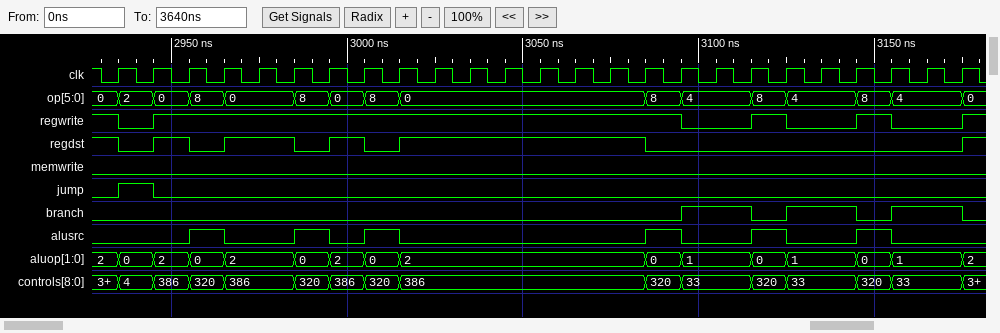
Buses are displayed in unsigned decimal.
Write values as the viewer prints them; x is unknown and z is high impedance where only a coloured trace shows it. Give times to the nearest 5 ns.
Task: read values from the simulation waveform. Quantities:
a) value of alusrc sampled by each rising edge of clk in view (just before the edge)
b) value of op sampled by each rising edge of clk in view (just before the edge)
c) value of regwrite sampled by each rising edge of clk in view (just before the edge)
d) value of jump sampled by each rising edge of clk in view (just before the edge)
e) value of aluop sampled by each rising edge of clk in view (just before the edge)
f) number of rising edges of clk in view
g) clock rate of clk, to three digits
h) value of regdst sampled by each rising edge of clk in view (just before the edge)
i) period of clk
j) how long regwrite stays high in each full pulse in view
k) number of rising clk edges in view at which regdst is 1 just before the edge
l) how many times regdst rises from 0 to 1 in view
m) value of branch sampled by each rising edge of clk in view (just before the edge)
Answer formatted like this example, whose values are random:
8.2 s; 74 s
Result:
0 0 0 1 0 0 1 0 1 0 0 0 0 0 0 0 1 0 0 1 0 0 1 0 0; 0, 2, 0, 8, 0, 0, 8, 0, 8, 0, 0, 0, 0, 0, 0, 0, 8, 4, 4, 8, 4, 4, 8, 4, 4; 1 0 1 1 1 1 1 1 1 1 1 1 1 1 1 1 1 0 0 1 0 0 1 0 0; 0 1 0 0 0 0 0 0 0 0 0 0 0 0 0 0 0 0 0 0 0 0 0 0 0; 2, 0, 2, 0, 2, 2, 0, 2, 0, 2, 2, 2, 2, 2, 2, 2, 0, 1, 1, 0, 1, 1, 0, 1, 1; 25; 100 MHz; 1 0 1 0 1 1 0 1 0 1 1 1 1 1 1 1 0 0 0 0 0 0 0 0 0; 10 ns; 150 ns, 10 ns, 10 ns; 12; 5; 0 0 0 0 0 0 0 0 0 0 0 0 0 0 0 0 0 1 1 0 1 1 0 1 1
